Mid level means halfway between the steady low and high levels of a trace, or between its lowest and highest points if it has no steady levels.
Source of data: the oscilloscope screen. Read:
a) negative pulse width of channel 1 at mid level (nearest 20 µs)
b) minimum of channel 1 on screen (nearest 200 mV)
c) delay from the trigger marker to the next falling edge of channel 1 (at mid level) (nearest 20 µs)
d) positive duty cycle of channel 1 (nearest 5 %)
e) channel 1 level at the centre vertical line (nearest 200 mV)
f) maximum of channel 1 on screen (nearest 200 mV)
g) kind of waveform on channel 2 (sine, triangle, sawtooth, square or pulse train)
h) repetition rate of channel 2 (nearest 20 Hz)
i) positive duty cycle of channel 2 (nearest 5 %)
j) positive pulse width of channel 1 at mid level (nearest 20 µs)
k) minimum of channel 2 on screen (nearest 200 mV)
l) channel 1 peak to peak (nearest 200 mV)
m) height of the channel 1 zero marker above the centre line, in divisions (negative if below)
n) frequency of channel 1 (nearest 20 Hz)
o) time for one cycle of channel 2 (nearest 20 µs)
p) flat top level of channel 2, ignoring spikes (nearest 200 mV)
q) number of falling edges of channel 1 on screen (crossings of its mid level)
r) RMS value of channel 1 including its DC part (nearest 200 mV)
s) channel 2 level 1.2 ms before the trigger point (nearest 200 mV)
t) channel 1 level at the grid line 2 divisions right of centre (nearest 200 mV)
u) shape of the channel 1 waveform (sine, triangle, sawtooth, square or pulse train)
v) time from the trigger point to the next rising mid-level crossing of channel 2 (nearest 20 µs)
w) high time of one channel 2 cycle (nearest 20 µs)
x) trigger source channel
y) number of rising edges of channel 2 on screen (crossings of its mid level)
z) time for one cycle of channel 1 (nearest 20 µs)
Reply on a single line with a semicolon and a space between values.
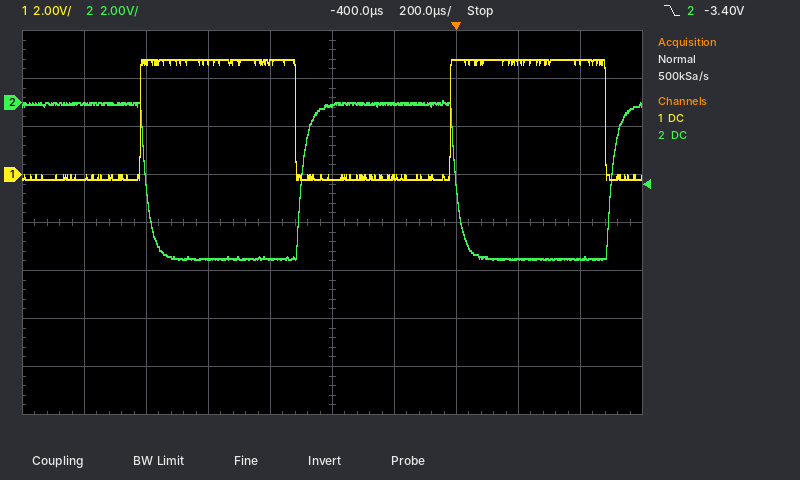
500 µs; -200 mV; 480 µs; 50 %; -200 mV; 4.8 V; square; 1.00 kHz; 50 %; 500 µs; -6.6 V; 5.0 V; +1.0 div; 1.00 kHz; 1.00 ms; 0.0 V; 2; 3.4 V; 0.0 V; 4.8 V; square; 500 µs; 500 µs; channel 2; 2; 1.00 ms
